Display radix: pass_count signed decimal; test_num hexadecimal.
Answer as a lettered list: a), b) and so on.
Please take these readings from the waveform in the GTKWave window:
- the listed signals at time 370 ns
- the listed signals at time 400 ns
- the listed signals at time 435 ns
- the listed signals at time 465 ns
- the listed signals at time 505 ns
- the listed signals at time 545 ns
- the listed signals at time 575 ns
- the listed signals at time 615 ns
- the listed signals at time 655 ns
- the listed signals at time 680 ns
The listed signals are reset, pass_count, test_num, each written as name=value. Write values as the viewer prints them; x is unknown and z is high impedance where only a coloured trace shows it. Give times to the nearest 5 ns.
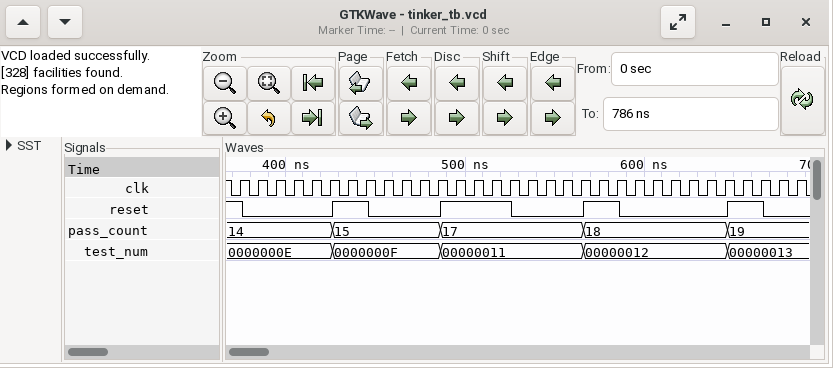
a) reset=1, pass_count=14, test_num=0000000E
b) reset=0, pass_count=14, test_num=0000000E
c) reset=1, pass_count=15, test_num=0000000F
d) reset=0, pass_count=15, test_num=0000000F
e) reset=1, pass_count=17, test_num=00000011
f) reset=0, pass_count=17, test_num=00000011
g) reset=1, pass_count=18, test_num=00000012
h) reset=0, pass_count=18, test_num=00000012
i) reset=1, pass_count=19, test_num=00000013
j) reset=0, pass_count=19, test_num=00000013
